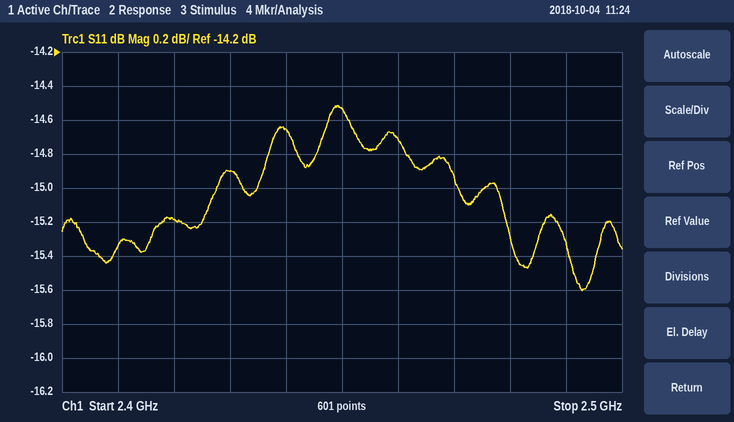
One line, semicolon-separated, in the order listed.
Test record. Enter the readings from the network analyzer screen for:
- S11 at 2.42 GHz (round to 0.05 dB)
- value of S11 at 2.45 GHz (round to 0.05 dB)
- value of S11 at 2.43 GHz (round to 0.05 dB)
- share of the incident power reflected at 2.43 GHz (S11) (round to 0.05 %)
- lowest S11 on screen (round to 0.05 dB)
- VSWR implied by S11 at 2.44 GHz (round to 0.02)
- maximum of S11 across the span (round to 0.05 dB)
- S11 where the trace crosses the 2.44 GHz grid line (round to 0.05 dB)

-15.20 dB; -14.55 dB; -14.90 dB; 3.25 %; -15.60 dB; 1.46; -14.50 dB; -14.65 dB
